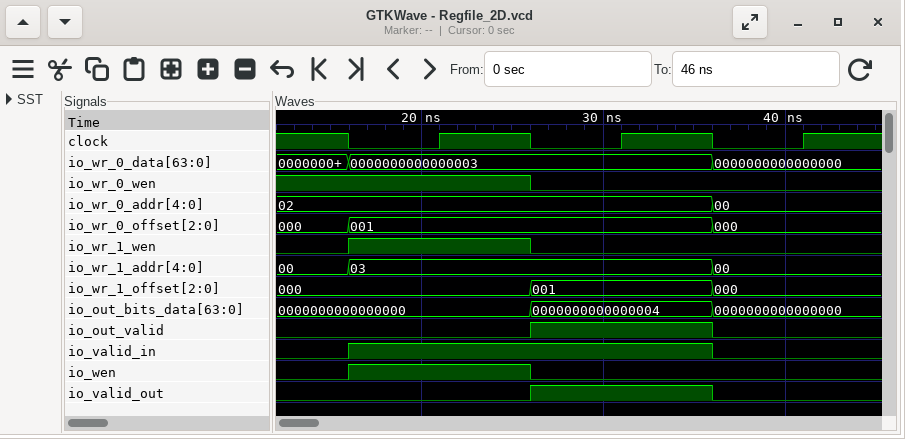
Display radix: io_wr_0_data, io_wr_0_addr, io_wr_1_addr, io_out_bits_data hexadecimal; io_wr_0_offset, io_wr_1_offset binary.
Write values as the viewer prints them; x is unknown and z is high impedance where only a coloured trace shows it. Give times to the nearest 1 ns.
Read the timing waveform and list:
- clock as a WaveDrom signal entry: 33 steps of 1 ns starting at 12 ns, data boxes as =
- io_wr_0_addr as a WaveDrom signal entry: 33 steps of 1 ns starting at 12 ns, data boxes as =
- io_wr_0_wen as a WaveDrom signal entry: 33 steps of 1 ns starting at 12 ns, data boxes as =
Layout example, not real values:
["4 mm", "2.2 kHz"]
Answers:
["{name: 'clock', wave: '1...0....1....0....1....0....1...'}", "{name: 'io_wr_0_addr', wave: '=.......................=........', data: '02 00'}", "{name: 'io_wr_0_wen', wave: '1.............0..................'}"]
